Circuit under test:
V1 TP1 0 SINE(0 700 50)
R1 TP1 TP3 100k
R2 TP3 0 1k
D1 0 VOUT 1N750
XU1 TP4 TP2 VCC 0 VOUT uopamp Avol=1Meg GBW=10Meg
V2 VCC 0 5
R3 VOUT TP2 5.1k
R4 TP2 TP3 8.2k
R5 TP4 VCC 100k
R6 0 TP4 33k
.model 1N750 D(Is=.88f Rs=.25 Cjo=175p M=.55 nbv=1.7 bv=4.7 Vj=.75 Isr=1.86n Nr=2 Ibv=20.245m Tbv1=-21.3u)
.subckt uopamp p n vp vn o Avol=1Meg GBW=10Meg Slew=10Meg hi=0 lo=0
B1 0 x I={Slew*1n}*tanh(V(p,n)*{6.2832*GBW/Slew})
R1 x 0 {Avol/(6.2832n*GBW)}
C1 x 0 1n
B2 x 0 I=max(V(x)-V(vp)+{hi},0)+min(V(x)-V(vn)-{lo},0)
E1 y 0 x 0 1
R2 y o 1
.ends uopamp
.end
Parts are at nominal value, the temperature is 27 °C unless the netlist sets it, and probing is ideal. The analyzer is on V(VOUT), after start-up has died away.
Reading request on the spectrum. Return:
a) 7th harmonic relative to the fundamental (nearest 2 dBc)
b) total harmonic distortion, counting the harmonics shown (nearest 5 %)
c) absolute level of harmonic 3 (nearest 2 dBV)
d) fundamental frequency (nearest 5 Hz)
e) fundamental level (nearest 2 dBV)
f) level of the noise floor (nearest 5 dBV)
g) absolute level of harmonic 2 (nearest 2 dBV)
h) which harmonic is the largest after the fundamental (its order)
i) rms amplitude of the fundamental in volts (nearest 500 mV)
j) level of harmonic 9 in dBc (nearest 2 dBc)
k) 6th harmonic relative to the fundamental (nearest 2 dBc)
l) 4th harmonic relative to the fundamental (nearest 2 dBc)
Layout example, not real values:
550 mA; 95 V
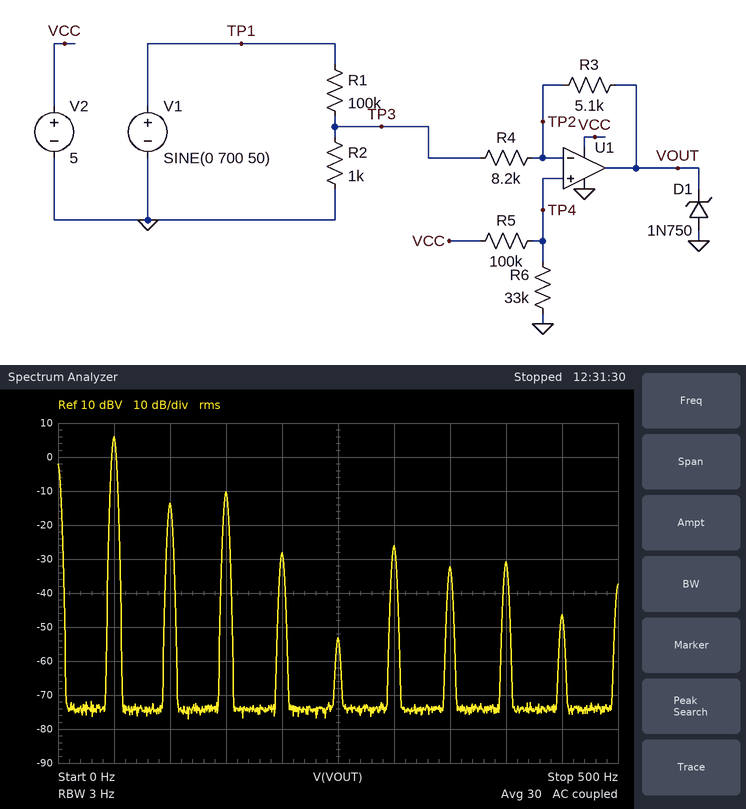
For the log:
-38 dBc; 20 %; -10 dBV; 50 Hz; 6 dBV; -75 dBV; -14 dBV; 3; 2.0 V; -52 dBc; -32 dBc; -34 dBc
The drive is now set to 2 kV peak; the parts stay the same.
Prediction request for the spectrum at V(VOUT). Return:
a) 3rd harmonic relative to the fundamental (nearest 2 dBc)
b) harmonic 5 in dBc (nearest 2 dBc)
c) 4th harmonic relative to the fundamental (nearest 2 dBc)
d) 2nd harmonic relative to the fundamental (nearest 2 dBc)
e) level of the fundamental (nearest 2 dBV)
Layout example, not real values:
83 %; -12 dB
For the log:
-10 dBc; -16 dBc; -28 dBc; -28 dBc; 6 dBV
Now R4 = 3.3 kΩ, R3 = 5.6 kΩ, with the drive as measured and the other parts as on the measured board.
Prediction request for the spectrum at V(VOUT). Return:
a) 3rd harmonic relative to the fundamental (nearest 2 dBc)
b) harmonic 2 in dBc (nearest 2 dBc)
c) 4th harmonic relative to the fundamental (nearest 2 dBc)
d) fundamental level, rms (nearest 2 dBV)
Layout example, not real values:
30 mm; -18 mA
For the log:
-10 dBc; -26 dBc; -28 dBc; 6 dBV
